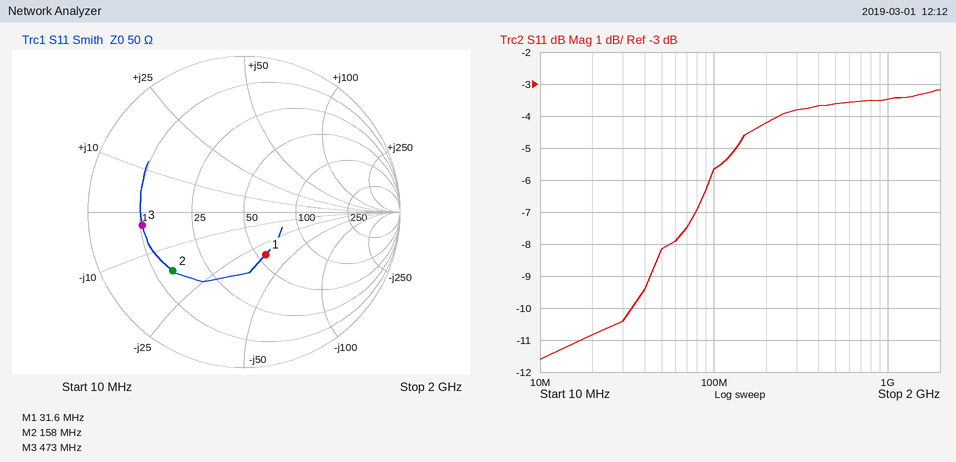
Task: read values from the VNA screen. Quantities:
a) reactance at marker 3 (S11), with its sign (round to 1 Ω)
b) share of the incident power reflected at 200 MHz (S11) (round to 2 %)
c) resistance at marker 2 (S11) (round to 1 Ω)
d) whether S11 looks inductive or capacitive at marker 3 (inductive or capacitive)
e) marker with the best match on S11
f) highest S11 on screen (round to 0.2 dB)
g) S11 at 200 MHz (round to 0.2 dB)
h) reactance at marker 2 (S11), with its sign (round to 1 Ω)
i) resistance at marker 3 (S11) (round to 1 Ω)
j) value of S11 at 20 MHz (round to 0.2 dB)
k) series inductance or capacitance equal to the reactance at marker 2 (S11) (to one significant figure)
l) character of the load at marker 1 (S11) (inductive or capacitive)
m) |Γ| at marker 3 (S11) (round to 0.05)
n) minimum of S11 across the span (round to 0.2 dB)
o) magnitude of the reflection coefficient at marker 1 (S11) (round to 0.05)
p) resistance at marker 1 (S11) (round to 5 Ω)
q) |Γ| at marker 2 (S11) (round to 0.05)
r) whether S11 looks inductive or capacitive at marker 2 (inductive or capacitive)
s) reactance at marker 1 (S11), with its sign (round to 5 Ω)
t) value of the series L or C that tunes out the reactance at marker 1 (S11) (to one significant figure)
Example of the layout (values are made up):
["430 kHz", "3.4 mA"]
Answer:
["-3 Ω", "38 %", "14 Ω", "capacitive", "marker 1", "-3.2 dB", "-4.2 dB", "-17 Ω", "10 Ω", "-10.8 dB", "60 pF", "capacitive", "0.65", "-11.6 dB", "0.30", "55 Ω", "0.60", "capacitive", "-35 Ω", "200 nH"]
